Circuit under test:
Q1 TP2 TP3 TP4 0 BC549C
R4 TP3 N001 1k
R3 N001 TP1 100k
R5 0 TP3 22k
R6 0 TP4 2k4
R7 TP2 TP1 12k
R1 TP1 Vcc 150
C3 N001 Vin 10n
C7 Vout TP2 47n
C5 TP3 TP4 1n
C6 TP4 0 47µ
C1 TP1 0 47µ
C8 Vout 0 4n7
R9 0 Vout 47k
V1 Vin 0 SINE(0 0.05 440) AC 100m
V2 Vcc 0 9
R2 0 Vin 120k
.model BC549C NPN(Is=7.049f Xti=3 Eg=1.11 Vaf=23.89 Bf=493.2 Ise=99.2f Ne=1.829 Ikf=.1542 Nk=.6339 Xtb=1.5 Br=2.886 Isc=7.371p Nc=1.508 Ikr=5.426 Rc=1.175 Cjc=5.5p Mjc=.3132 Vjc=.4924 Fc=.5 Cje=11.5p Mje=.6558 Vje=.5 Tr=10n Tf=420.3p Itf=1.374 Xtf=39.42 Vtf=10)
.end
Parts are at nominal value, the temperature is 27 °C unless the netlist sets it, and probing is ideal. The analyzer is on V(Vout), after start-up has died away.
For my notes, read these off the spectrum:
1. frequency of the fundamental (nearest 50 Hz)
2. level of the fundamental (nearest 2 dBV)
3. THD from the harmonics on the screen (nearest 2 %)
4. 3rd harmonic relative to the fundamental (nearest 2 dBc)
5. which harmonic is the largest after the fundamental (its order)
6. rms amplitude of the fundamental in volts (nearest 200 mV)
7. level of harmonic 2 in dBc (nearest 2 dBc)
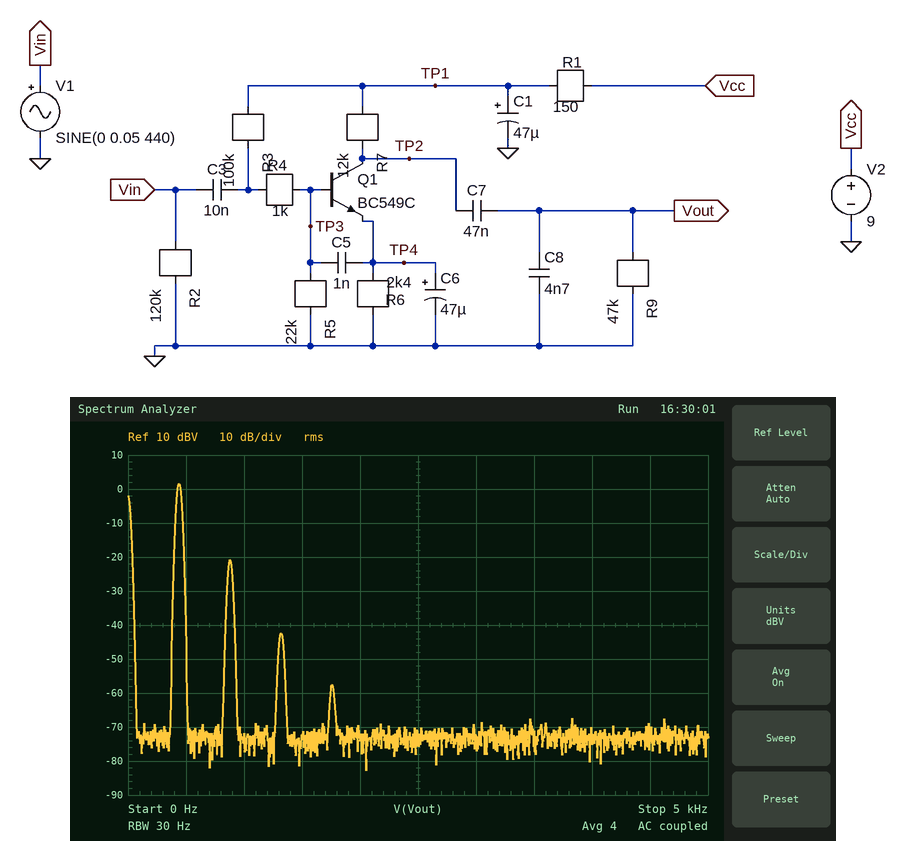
450 Hz
2 dBV
8 %
-44 dBc
2
1.2 V
-22 dBc
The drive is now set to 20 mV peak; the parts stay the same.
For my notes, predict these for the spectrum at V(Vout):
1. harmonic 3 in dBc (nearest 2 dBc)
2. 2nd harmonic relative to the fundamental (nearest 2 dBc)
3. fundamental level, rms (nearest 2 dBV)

-60 dBc
-30 dBc
-6 dBV
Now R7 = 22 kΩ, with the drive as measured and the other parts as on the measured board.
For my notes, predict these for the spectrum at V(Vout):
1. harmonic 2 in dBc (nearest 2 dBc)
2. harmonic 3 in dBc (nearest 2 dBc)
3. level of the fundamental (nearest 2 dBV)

-20 dBc
-38 dBc
-42 dBV
